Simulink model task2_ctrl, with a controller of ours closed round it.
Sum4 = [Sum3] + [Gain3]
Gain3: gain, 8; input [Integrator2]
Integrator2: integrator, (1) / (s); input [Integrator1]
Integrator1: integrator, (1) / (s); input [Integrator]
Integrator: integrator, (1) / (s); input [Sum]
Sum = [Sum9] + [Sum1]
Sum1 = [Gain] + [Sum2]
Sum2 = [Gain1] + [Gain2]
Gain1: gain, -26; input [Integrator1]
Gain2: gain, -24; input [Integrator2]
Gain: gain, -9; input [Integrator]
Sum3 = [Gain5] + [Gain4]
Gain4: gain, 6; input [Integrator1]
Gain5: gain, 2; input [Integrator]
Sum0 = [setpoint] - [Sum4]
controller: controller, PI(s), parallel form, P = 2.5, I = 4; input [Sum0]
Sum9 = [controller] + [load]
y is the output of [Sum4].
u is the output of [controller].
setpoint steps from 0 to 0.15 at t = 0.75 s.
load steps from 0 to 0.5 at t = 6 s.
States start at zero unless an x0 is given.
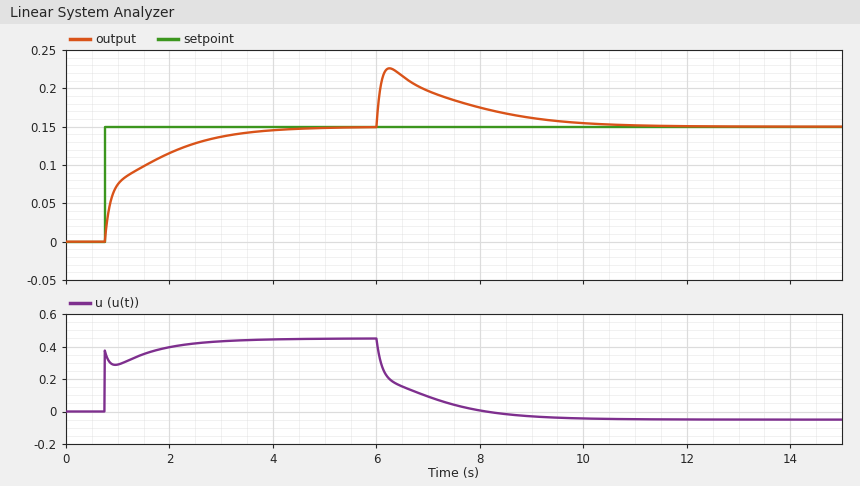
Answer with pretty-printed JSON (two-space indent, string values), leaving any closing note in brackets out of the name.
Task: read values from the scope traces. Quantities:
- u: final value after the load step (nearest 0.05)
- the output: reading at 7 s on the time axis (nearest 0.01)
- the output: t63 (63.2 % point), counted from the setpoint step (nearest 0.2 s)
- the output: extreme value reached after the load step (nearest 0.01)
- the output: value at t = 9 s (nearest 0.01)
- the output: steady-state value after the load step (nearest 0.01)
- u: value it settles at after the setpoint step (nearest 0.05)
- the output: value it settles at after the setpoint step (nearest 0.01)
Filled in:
{
  "u: final value after the load step": "-0.05",
  "the output: reading at 7 s on the time axis": "0.20",
  "the output: t63 (63.2 % point), counted from the setpoint step": "0.6 s",
  "the output: extreme value reached after the load step": "0.23",
  "the output: value at t = 9 s": "0.16",
  "the output: steady-state value after the load step": "0.15",
  "u: value it settles at after the setpoint step": "0.45",
  "the output: value it settles at after the setpoint step": "0.15"
}
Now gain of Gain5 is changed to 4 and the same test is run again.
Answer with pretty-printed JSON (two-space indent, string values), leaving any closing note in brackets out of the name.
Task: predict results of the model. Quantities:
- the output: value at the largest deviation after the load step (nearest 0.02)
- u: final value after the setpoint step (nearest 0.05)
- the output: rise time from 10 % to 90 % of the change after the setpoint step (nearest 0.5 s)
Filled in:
{
  "the output: value at the largest deviation after the load step": "0.24",
  "u: final value after the setpoint step": "0.45",
  "the output: rise time from 10 % to 90 % of the change after the setpoint step": "2.5 s"
}
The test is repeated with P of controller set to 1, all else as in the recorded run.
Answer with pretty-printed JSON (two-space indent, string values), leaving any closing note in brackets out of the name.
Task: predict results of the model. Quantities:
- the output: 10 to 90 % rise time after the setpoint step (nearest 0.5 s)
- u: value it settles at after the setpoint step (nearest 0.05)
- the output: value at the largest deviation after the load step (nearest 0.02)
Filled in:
{
  "the output: 10 to 90 % rise time after the setpoint step": "2.0 s",
  "u: value it settles at after the setpoint step": "0.45",
  "the output: value at the largest deviation after the load step": "0.24"
}
